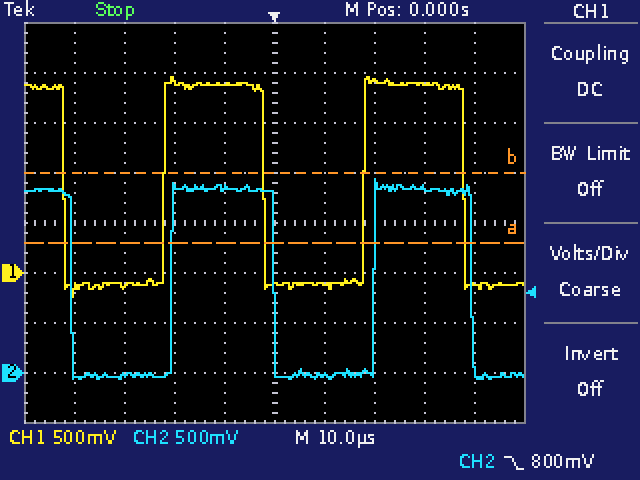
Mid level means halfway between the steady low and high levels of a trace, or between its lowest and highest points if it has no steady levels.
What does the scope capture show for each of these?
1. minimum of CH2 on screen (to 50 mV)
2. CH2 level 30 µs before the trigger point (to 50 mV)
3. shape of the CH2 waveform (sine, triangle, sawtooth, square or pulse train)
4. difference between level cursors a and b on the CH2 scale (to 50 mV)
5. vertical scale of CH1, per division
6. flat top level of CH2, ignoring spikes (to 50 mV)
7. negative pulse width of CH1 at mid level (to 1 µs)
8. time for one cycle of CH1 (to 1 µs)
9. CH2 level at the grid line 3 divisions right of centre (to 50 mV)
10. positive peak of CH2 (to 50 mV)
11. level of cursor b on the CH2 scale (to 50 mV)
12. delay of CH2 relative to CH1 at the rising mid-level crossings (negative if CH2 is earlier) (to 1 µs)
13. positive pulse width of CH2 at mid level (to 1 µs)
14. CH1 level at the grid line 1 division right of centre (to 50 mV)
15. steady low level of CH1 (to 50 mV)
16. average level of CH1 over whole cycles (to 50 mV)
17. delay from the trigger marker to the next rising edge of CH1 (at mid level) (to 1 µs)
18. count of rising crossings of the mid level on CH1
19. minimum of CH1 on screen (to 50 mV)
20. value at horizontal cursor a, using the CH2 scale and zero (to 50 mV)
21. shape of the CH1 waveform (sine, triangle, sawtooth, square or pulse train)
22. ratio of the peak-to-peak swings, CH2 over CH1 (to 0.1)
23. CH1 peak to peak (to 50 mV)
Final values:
-50 mV
-50 mV
square
700 mV
500 mV
1.85 V
20 µs
40 µs
1.85 V
1.95 V
2.00 V
+2 µs
20 µs
-100 mV
-100 mV
900 mV
18 µs
2
-250 mV
1.30 V
square
0.9
2.20 V
